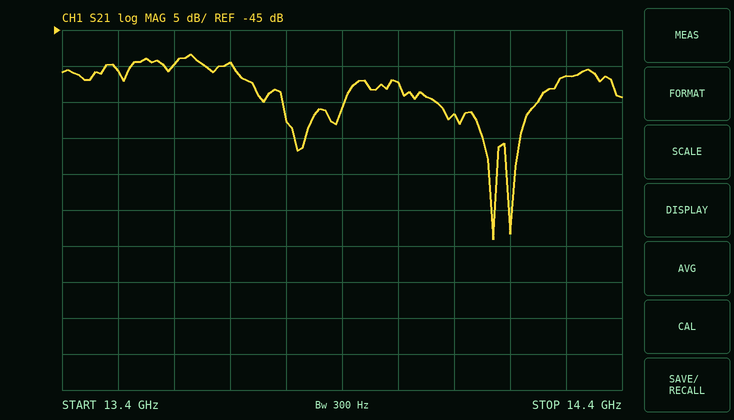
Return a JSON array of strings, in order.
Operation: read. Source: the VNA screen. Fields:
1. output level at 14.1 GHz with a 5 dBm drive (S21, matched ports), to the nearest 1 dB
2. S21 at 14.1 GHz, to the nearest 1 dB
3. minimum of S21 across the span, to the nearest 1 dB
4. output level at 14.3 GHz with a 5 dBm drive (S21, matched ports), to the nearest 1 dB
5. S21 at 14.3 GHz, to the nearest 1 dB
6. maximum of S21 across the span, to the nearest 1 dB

["-52 dBm", "-57 dB", "-74 dB", "-46 dBm", "-51 dB", "-48 dB"]
